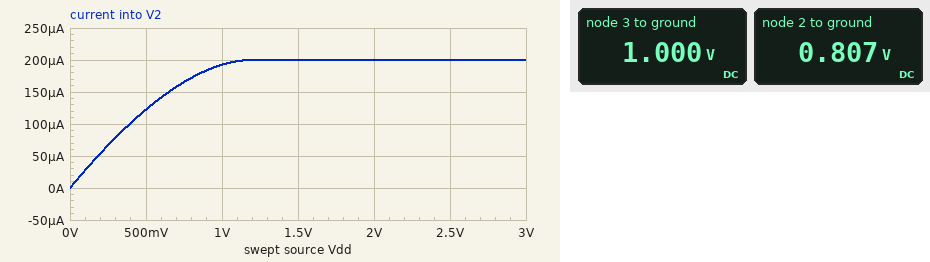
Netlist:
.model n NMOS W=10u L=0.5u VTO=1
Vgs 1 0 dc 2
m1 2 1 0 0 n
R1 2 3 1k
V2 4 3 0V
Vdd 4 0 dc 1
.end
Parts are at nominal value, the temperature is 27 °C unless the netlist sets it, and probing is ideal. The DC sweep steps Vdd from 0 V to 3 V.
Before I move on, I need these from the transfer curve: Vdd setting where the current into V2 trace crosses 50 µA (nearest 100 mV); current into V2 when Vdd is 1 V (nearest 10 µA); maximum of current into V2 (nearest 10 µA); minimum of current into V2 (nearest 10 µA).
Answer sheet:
200 mV
190 µA
200 µA
0 A
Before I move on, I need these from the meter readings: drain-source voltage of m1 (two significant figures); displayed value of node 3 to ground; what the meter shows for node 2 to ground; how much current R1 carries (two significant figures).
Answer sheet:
810 mV
1.000 V
0.807 V
190 µA
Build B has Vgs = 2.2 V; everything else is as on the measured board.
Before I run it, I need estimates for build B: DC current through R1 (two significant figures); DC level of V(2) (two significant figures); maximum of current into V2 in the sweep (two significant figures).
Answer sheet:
250 µA
750 mV
290 µA
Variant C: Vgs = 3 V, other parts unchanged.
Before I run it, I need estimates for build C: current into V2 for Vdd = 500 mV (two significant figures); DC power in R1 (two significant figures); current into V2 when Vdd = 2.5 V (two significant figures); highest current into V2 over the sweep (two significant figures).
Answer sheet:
210 µA
160 µW
780 µA
800 µA
